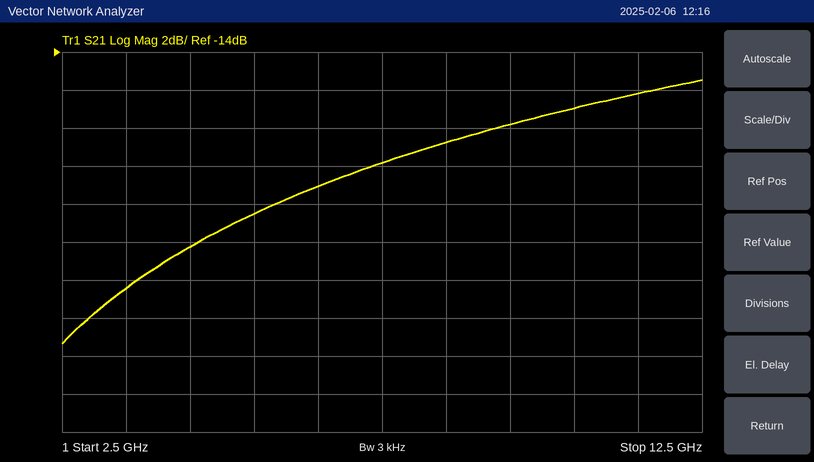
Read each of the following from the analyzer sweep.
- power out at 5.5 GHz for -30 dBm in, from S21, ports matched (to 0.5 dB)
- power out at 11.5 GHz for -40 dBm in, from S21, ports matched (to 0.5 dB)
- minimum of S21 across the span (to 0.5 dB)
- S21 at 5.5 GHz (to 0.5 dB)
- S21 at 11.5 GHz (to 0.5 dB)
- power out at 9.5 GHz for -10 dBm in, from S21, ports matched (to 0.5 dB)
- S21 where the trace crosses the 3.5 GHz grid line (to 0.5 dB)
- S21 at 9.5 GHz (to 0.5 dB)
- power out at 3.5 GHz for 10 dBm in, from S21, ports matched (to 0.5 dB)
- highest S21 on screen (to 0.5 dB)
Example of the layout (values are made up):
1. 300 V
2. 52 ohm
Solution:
1. -52.5 dBm
2. -56.0 dBm
3. -29.5 dB
4. -22.5 dB
5. -16.0 dB
6. -28.0 dBm
7. -26.5 dB
8. -18.0 dB
9. -16.5 dBm
10. -15.5 dB
